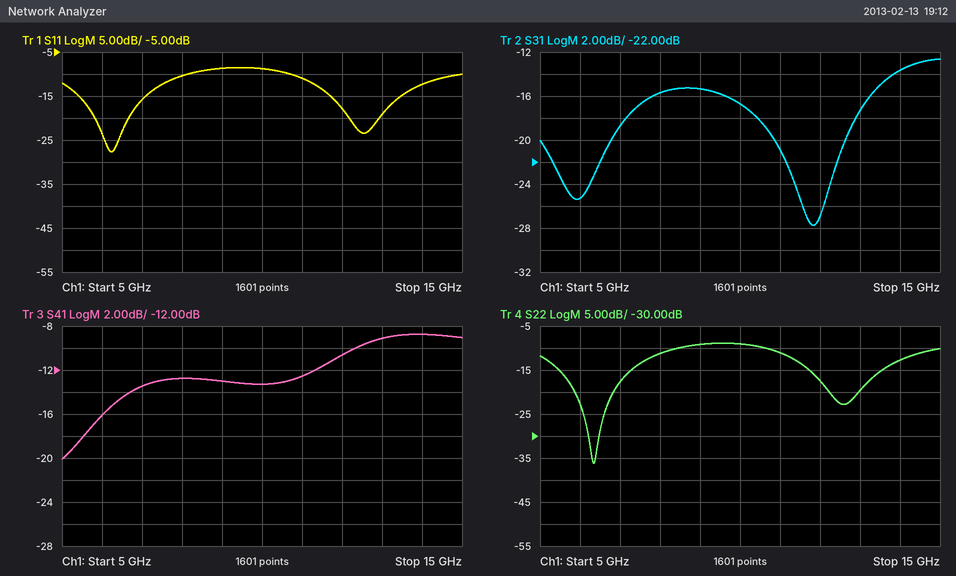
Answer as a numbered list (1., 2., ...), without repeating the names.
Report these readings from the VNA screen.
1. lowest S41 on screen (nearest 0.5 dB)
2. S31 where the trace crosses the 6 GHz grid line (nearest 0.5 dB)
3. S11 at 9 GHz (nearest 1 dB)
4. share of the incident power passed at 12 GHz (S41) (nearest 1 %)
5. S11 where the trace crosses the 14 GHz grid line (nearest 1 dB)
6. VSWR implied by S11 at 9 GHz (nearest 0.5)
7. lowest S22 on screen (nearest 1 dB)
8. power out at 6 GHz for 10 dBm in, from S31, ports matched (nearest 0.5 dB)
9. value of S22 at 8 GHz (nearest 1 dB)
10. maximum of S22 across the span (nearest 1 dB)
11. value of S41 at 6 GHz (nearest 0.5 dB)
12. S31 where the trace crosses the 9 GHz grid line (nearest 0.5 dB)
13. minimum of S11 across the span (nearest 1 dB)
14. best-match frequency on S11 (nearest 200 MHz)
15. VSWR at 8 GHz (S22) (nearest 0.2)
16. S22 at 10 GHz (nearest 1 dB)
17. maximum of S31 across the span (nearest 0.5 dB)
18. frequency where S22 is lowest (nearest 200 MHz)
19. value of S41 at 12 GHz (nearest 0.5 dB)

1. -20.0 dB
2. -25.5 dB
3. -9 dB
4. 9 %
5. -12 dB
6. 2.0
7. -36 dB
8. -15.5 dBm
9. -11 dB
10. -9 dB
11. -16.0 dB
12. -15.5 dB
13. -28 dB
14. 6.2 GHz
15. 1.8
16. -9 dB
17. -12.5 dB
18. 6.4 GHz
19. -10.5 dB
